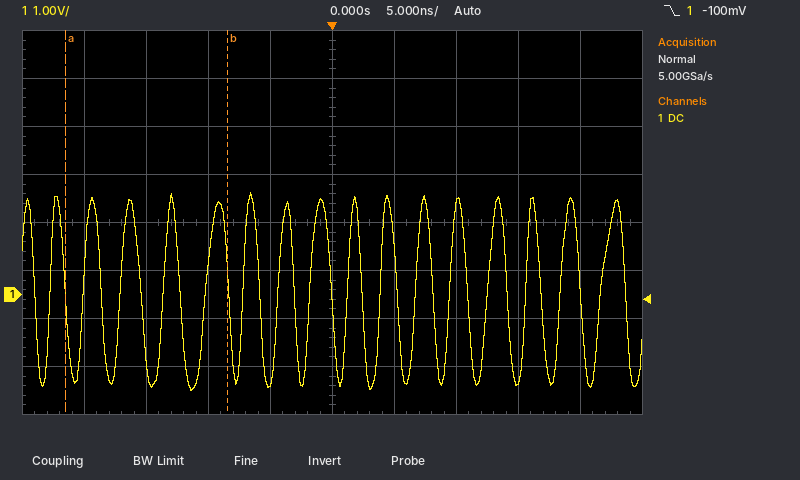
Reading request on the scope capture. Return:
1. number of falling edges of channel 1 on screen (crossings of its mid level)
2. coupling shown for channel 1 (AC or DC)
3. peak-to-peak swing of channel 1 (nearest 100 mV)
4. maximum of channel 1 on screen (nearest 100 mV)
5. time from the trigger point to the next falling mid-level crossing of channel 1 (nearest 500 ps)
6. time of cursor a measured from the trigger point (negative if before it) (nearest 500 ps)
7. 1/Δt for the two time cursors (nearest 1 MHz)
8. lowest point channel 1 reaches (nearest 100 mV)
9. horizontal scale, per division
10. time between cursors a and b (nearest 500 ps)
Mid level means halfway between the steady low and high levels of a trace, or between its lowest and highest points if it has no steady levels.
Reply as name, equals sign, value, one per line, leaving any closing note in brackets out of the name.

number of falling edges of channel 1 on screen = 17
coupling shown for channel 1 = DC
peak-to-peak swing of channel 1 = 4.1 V
maximum of channel 1 on screen = 2.1 V
time from the trigger point to the next falling mid-level crossing of channel 1 = 2.5 ns
time of cursor a measured from the trigger point (negative if before it) = -21.5 ns
1/Δt for the two time cursors = 77 MHz
lowest point channel 1 reaches = -2.0 V
horizontal scale, per division = 5 ns
time between cursors a and b = 13.0 ns
